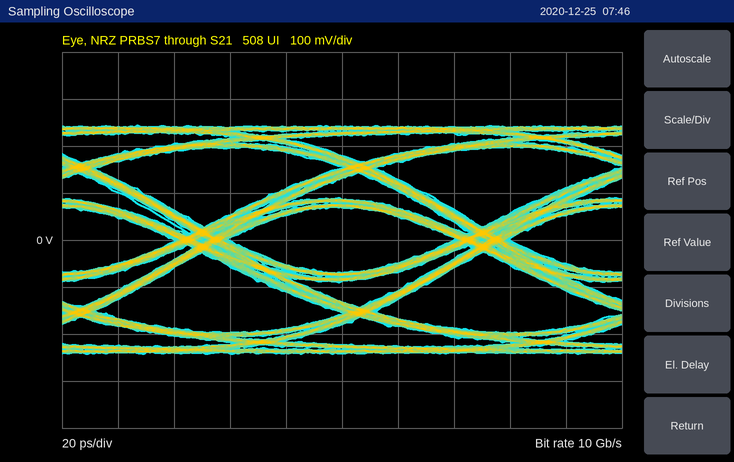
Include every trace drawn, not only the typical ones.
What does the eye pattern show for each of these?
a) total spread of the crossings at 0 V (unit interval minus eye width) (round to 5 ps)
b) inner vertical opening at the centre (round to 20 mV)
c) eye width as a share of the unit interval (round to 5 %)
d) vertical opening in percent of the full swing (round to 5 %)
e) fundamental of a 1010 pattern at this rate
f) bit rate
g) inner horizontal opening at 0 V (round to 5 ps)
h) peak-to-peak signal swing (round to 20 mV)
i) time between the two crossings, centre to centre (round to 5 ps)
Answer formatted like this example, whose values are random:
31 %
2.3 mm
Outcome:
20 ps
140 mV
80 %
30 %
5 GHz
10 Gb/s
80 ps
480 mV
100 ps
